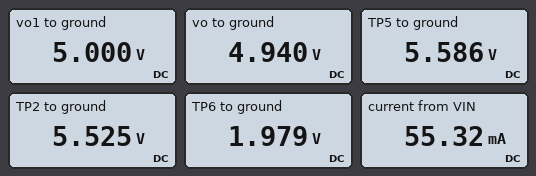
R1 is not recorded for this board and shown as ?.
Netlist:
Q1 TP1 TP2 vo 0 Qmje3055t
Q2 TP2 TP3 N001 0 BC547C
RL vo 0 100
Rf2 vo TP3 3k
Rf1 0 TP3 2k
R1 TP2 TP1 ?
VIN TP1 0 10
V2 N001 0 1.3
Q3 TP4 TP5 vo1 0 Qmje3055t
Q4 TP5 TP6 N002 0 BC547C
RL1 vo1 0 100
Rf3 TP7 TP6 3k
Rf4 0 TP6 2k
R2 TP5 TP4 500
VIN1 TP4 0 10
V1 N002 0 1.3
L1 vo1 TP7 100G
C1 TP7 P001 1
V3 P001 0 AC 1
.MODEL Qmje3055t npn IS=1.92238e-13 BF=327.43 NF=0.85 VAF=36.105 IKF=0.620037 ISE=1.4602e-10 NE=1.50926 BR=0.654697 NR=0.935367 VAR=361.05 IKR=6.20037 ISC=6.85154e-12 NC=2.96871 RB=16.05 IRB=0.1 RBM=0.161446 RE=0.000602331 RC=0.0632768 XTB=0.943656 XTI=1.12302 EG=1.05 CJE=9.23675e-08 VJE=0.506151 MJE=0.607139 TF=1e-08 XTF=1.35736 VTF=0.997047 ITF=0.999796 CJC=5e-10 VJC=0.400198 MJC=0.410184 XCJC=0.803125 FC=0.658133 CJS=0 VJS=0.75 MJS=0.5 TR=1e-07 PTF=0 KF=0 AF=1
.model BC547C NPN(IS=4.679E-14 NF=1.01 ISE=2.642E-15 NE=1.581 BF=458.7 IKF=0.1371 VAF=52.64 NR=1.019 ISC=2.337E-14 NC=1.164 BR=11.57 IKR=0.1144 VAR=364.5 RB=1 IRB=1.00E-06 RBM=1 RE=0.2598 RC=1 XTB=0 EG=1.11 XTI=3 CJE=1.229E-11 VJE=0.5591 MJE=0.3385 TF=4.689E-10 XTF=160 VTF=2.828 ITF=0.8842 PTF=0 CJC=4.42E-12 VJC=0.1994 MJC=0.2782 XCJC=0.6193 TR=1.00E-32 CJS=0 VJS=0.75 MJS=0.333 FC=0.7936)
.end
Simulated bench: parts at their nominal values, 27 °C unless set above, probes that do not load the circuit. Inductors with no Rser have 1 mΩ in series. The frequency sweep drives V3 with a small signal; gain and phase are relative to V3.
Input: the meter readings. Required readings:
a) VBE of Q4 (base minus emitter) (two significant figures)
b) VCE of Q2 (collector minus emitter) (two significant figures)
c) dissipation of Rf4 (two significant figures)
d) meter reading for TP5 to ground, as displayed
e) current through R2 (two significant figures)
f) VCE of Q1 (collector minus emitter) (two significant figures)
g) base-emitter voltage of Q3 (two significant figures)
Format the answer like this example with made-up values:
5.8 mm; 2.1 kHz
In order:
680 mV; 4.2 V; 2.0 mW; 5.586 V; 8.8 mA; 5.1 V; 590 mV
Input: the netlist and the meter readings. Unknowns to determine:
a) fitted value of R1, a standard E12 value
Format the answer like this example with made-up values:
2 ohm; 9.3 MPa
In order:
820 Ω
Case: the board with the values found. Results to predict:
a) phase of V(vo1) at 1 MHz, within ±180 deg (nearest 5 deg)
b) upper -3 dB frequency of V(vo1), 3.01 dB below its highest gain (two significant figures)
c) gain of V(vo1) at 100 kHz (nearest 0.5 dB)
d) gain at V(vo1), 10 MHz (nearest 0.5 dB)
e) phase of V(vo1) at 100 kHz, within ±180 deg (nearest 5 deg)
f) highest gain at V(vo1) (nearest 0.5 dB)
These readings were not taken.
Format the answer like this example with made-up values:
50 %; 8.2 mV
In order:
100 deg; 130 kHz; 27.0 dB; -8.0 dB; 145 deg; 29.0 dB
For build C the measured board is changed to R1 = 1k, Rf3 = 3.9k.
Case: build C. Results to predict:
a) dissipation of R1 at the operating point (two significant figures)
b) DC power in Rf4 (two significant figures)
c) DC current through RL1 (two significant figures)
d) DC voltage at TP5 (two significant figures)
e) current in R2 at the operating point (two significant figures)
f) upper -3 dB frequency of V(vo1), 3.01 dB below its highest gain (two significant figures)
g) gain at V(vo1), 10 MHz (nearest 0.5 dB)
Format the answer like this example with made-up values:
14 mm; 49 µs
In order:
20 mW; 1.9 mW; 59 mA; 6.5 V; 7.1 mA; 140 kHz; -11.0 dB
